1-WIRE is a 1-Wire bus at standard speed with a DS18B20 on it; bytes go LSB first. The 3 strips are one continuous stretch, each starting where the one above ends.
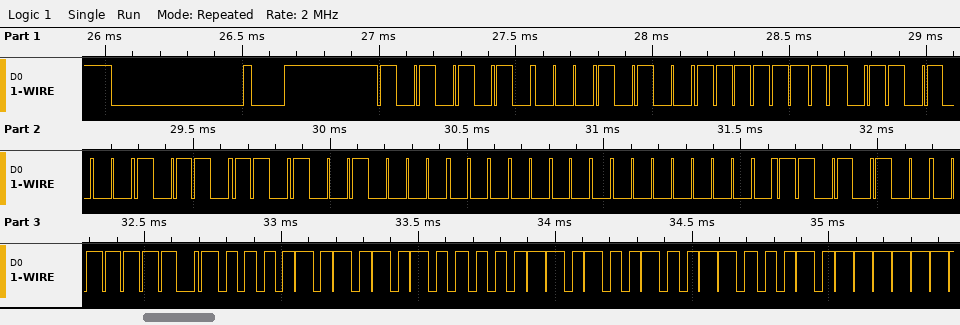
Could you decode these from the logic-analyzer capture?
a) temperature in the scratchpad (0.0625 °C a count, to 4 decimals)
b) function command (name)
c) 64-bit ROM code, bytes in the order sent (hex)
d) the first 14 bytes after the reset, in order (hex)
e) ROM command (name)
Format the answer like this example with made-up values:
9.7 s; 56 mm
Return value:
85.0000 °C; Read Scratchpad; 28 FF 16 6D 09 00 00 2B; 55 28 FF 16 6D 09 00 00 2B BE 50 05 4B 46; Match ROM
